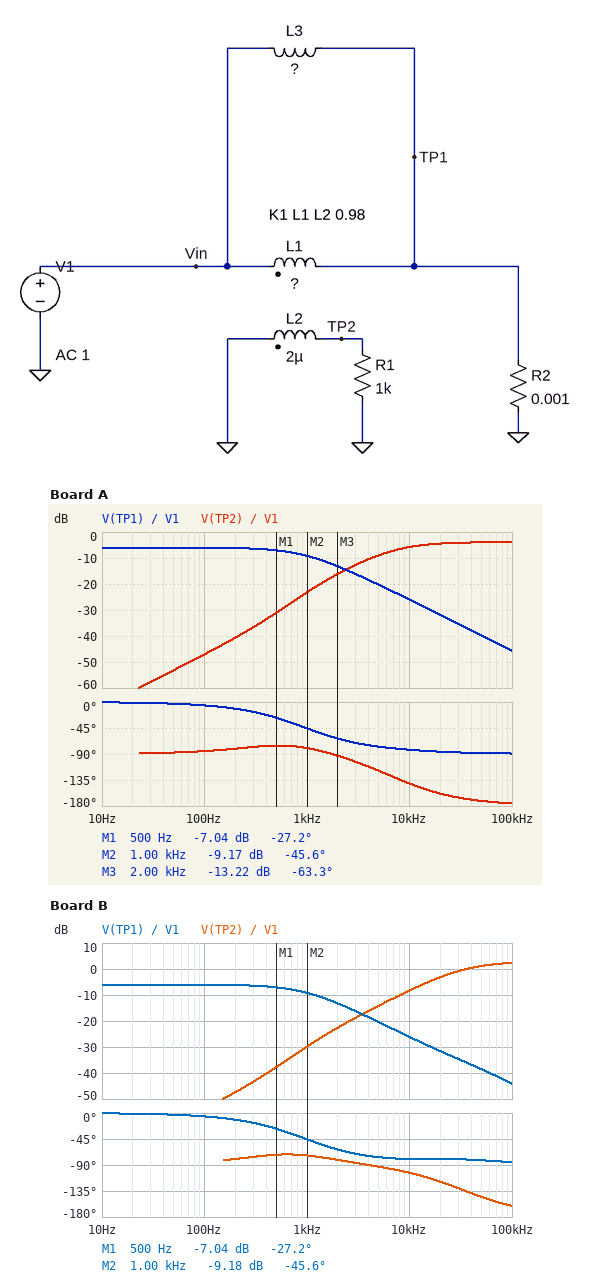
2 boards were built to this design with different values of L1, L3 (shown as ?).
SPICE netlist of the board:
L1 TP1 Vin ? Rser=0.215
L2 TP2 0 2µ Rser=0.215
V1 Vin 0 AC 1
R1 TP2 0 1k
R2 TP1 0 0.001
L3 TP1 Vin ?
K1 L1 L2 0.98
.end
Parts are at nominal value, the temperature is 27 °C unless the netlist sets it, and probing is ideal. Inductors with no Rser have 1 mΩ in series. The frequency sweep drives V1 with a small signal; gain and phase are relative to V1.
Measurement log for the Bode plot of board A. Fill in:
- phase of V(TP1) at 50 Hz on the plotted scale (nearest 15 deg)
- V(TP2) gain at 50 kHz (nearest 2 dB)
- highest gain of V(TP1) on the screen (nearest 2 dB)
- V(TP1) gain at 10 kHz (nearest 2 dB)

0 deg
-4 dB
-6 dB
-26 dB
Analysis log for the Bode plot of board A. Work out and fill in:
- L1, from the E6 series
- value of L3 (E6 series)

4.7 µH
330 nH
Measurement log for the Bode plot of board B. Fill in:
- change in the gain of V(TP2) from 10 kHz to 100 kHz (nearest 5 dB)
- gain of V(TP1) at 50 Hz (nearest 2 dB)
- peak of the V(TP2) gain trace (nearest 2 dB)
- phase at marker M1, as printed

10 dB
-6 dB
2 dB
-27.2 deg
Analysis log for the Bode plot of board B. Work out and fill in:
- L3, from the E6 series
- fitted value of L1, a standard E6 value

330 nH
1 µH
